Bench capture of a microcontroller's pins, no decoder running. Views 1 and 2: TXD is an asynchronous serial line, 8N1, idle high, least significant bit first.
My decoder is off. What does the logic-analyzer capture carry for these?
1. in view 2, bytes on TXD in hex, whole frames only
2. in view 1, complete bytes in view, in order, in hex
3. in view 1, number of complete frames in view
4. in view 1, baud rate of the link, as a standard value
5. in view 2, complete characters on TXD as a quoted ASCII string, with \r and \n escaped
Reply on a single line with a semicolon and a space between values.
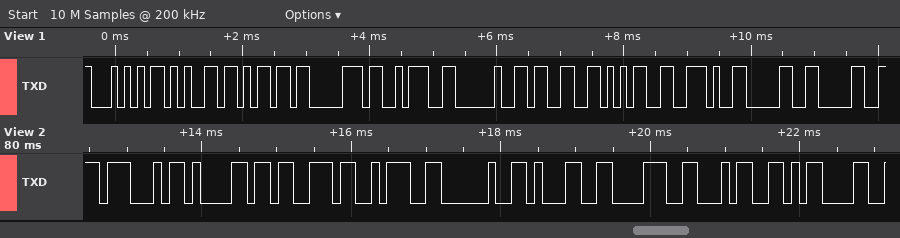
47 61 73 3A 20 31 38 34 0D; 0x54 0x65 0x6D 0x70 0x3A 0x20 0x33 0x35 0x2E 0x30 0x30; 11; 9600 baud; "Gas: 184\r"
